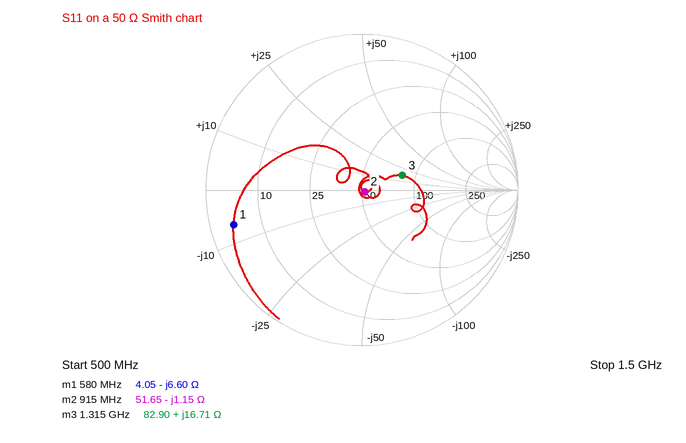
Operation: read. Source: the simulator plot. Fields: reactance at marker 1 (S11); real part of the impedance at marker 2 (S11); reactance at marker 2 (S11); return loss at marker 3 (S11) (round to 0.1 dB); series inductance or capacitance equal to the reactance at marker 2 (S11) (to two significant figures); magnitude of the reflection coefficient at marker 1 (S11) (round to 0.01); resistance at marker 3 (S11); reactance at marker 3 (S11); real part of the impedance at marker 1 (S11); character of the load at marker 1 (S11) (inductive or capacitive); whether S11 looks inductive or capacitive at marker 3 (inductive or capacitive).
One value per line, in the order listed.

-6.60 Ω
51.65 Ω
-1.15 Ω
11.2 dB
150 pF
0.85
82.90 Ω
+16.71 Ω
4.05 Ω
capacitive
inductive
